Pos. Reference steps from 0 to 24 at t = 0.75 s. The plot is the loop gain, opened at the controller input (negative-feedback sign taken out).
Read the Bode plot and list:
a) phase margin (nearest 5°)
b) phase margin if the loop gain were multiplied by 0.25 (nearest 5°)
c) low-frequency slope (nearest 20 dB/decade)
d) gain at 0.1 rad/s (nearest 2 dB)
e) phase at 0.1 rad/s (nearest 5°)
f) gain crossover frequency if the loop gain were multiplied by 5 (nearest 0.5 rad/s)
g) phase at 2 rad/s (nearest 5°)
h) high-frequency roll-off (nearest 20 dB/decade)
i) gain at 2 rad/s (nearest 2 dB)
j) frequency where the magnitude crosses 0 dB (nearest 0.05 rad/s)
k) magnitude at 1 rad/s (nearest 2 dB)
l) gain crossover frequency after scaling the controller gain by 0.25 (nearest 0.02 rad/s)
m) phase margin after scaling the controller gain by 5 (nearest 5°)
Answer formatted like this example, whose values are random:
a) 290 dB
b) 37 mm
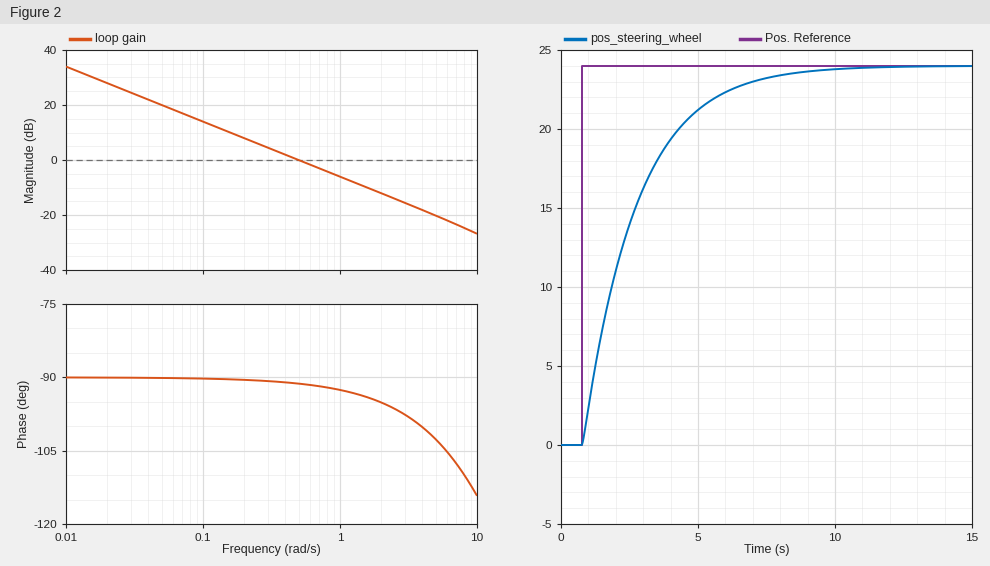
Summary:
a) 90°
b) 90°
c) -20 dB/decade
d) 14 dB
e) -90°
f) 2.5 rad/s
g) -95°
h) -20 dB/decade
i) -12 dB
j) 0.50 rad/s
k) -6 dB
l) 0.12 rad/s
m) 85°
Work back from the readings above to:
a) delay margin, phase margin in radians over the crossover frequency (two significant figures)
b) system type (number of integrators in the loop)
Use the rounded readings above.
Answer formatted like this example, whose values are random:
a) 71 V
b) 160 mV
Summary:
a) 3.1 s
b) 1
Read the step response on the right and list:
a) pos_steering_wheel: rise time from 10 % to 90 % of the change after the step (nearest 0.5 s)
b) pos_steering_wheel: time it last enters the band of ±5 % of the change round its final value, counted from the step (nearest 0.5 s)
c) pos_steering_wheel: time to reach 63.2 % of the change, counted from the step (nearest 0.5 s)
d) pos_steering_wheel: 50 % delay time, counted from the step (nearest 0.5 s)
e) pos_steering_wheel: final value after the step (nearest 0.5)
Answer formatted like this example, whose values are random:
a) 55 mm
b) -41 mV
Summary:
a) 4.5 s
b) 6.0 s
c) 2.0 s
d) 1.5 s
e) 24.0
